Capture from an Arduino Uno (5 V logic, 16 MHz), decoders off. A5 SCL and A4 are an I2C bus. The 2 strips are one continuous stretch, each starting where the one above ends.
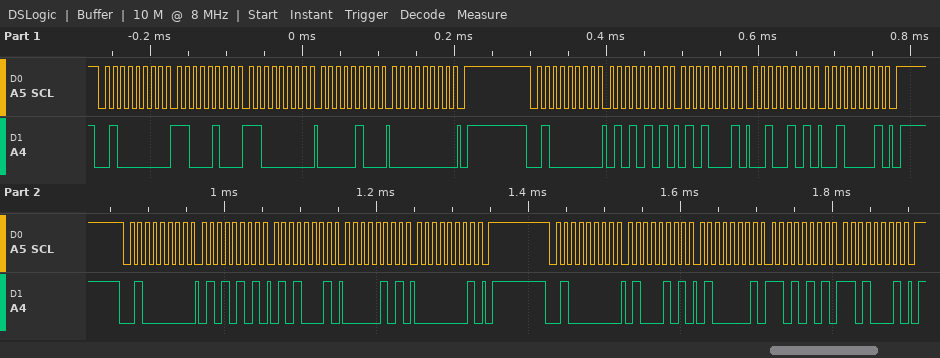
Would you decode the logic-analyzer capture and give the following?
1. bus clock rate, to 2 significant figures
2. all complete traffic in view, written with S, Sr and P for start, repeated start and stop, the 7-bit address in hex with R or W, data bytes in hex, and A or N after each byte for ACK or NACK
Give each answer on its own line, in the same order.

100 kHz
S 20W A C4 A C0 A 04 A 00 A P S 20W A 55 A 51 A 25 A 21 A P S 20W A 55 A 51 A 05 A 01 A P S 20W A 45 A 41 A D5 A D1 A P
